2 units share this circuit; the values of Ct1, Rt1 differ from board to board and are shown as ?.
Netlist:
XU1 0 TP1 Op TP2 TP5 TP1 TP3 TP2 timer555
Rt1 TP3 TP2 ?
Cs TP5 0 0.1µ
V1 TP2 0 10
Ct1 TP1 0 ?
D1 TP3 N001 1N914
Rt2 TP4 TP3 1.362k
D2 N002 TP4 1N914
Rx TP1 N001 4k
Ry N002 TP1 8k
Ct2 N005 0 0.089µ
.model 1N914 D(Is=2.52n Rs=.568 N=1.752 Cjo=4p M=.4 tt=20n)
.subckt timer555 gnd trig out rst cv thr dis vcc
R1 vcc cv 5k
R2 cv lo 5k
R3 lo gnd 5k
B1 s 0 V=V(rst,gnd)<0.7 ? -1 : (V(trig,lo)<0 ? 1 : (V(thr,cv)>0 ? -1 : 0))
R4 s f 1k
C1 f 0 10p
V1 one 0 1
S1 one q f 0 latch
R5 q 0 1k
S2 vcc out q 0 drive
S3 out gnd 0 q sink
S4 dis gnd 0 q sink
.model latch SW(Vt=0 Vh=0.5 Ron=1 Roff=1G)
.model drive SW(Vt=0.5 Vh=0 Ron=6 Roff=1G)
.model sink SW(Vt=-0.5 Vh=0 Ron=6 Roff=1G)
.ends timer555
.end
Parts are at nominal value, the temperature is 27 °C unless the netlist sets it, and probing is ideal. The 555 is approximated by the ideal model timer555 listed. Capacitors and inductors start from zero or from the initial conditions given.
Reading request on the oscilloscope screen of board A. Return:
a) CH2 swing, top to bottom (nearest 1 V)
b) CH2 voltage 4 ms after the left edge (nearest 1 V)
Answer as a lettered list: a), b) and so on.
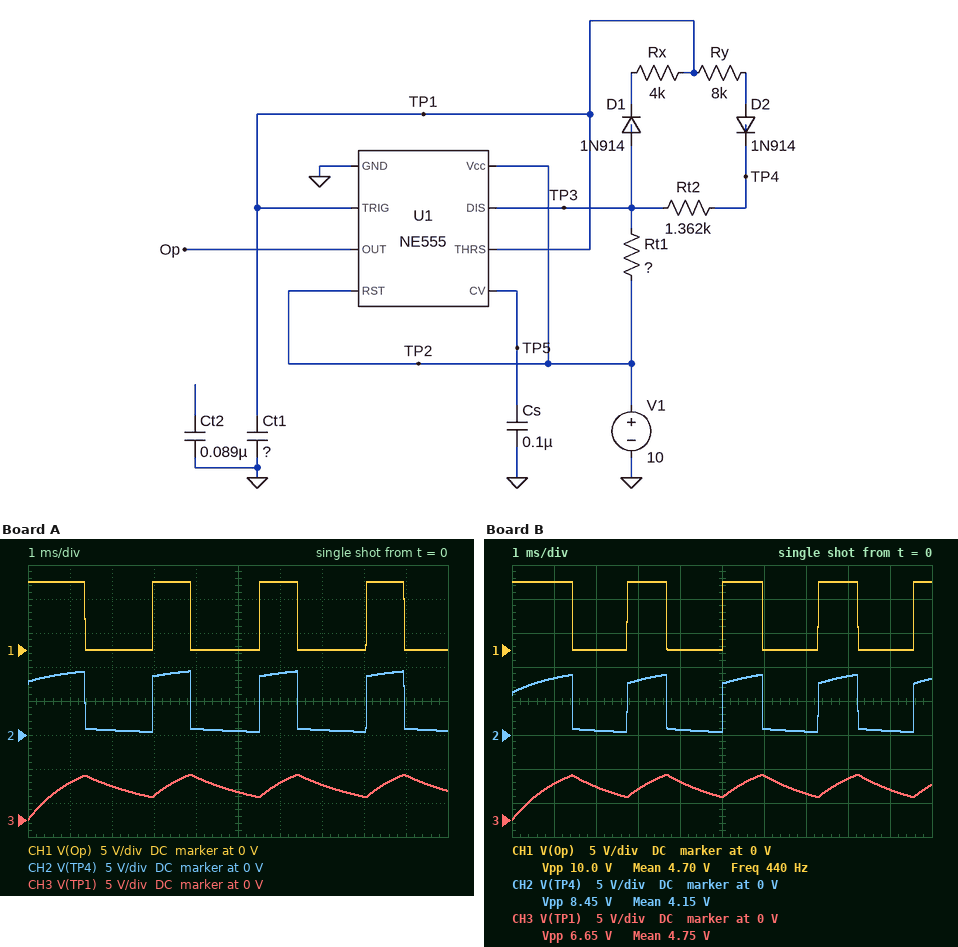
a) 9 V
b) 1 V
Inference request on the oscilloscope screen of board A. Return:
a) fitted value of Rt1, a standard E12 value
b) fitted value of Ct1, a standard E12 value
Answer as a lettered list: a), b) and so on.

a) 1.2 kΩ
b) 220 nF
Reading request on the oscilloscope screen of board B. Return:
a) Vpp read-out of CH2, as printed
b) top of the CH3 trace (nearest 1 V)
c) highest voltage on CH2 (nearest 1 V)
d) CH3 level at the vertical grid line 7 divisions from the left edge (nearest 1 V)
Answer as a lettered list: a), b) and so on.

a) 8.45 V
b) 7 V
c) 9 V
d) 4 V
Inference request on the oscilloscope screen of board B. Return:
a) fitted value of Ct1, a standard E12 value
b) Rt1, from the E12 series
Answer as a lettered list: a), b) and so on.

a) 180 nF
b) 2.7 kΩ
